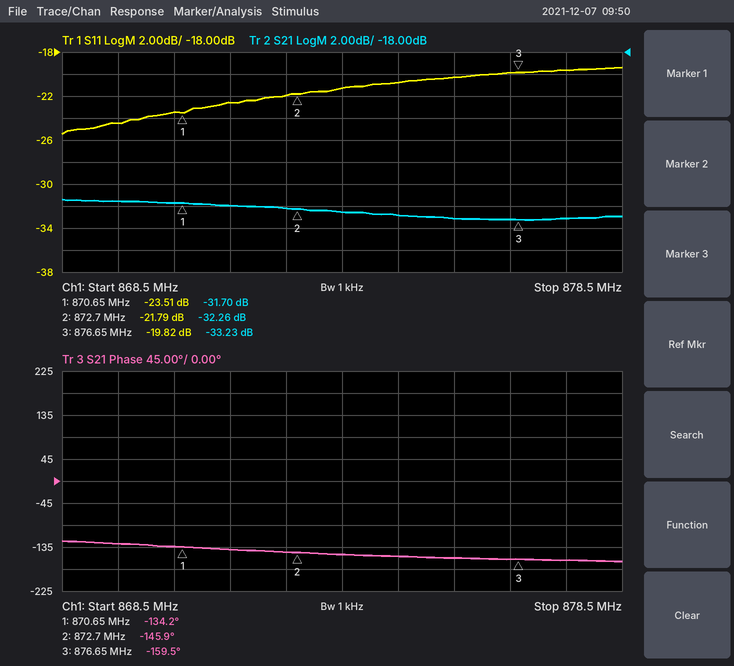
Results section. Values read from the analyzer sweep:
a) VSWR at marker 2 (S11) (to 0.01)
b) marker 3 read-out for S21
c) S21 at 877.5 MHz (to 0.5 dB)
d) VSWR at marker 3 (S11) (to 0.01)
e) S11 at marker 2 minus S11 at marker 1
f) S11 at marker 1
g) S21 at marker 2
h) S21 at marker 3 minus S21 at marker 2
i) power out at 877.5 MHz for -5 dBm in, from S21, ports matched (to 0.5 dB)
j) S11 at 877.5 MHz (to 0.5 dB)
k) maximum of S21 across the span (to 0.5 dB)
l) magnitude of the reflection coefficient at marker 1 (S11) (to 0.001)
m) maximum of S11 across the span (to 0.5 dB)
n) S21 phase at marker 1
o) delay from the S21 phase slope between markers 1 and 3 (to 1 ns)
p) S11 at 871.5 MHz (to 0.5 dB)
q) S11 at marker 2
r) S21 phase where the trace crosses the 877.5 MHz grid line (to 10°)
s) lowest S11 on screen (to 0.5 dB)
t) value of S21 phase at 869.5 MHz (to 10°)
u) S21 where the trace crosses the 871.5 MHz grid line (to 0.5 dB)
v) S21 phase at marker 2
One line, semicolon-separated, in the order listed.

1.18; -33.23 dB; -33.0 dB; 1.23; 1.72 dB; -23.51 dB; -32.26 dB; -0.97 dB; -38.0 dBm; -19.5 dB; -31.5 dB; 0.067; -19.5 dB; -134.2°; 12 ns; -22.5 dB; -21.79 dB; -160°; -25.5 dB; -130°; -32.0 dB; -145.9°
